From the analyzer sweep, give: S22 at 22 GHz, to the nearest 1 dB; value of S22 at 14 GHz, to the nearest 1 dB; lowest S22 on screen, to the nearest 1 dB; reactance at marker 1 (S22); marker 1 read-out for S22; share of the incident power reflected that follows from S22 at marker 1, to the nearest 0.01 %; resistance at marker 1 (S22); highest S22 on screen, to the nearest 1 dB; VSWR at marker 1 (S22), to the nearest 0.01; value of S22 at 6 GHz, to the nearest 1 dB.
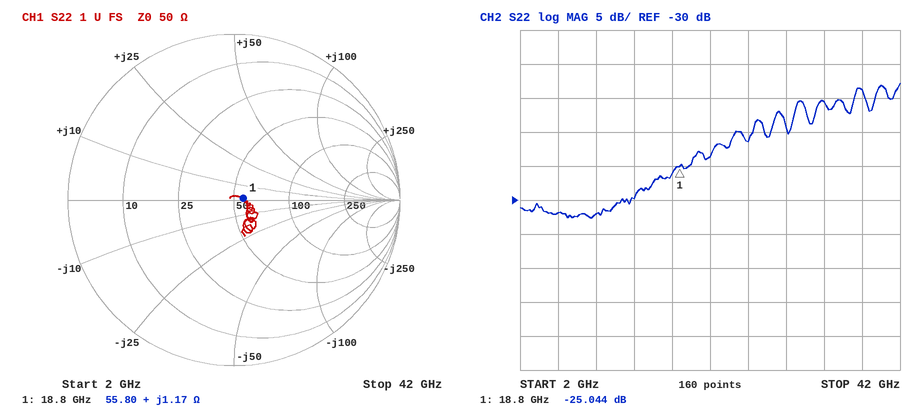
-24 dB
-30 dB
-33 dB
+1.17 Ω
-25.044 dB
0.31 %
55.80 Ω
-13 dB
1.12
-32 dB
